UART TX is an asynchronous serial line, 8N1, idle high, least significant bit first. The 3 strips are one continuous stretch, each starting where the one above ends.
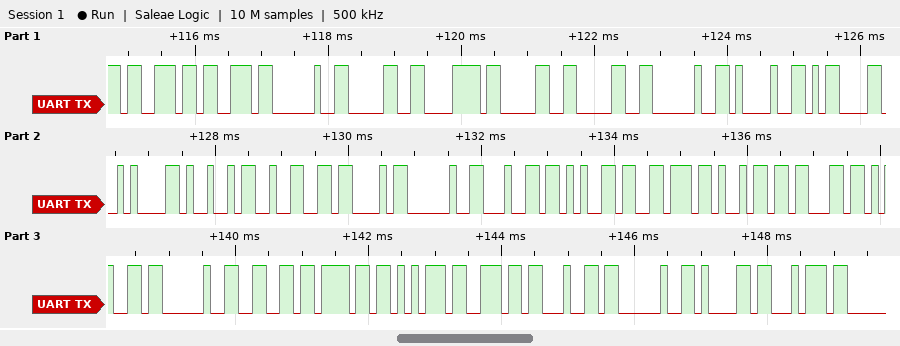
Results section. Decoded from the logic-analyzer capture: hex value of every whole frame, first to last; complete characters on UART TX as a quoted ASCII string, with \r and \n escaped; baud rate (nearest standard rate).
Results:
73 73 20 30 78 30 30 20 21 0D 0A 49 32 43 20 64 65 76 69 63 65 20 66 6F 75 6E 64 20 61 74
"ss 0x00 !\r\nI2C device found at"
9600 baud
